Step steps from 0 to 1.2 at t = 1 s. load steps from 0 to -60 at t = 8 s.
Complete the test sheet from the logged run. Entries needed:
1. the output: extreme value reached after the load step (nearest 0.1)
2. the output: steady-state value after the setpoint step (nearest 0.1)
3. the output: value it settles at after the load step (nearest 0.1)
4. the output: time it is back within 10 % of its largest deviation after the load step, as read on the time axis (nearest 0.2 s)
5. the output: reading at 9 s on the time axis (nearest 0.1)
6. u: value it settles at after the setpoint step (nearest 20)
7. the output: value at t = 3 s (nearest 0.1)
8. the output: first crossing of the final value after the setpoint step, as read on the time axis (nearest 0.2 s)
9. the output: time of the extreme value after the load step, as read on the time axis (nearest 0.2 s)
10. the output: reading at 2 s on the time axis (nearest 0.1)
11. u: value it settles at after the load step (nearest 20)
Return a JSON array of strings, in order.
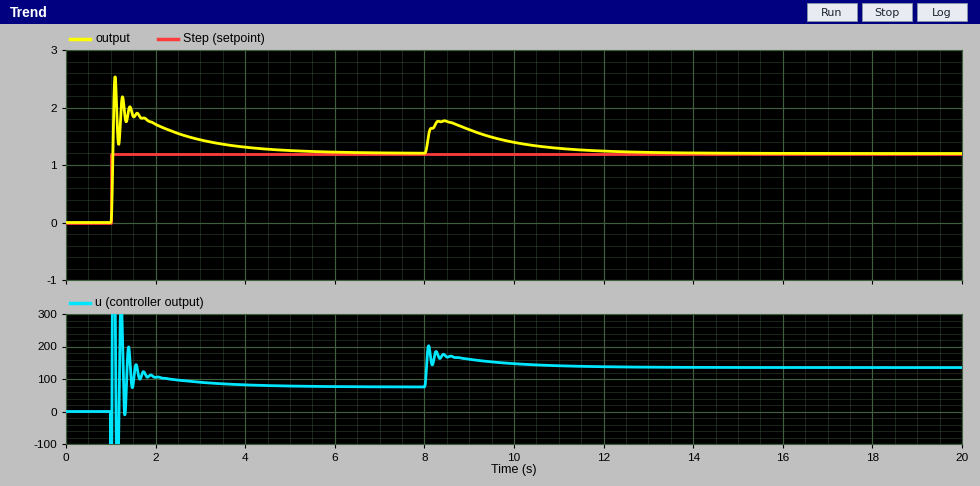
["1.8", "1.2", "1.2", "11.6 s", "1.6", "80", "1.4", "1.0 s", "8.4 s", "1.7", "140"]
